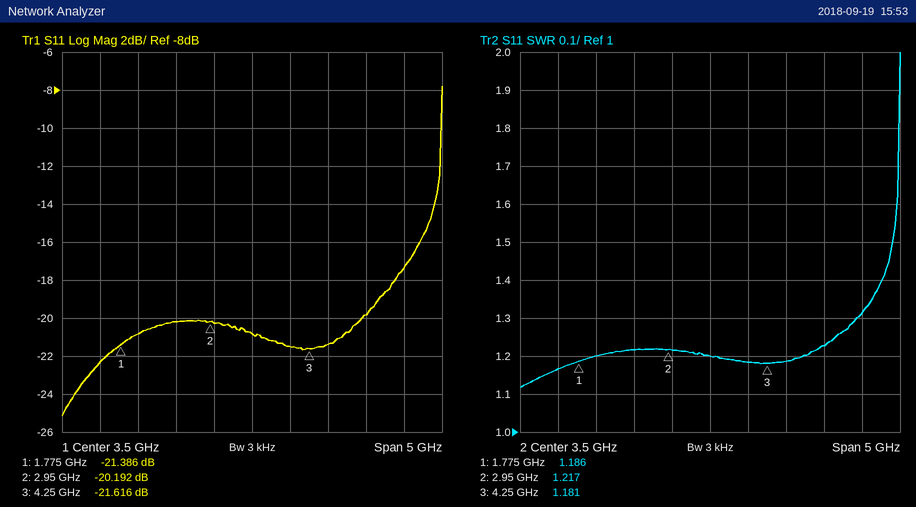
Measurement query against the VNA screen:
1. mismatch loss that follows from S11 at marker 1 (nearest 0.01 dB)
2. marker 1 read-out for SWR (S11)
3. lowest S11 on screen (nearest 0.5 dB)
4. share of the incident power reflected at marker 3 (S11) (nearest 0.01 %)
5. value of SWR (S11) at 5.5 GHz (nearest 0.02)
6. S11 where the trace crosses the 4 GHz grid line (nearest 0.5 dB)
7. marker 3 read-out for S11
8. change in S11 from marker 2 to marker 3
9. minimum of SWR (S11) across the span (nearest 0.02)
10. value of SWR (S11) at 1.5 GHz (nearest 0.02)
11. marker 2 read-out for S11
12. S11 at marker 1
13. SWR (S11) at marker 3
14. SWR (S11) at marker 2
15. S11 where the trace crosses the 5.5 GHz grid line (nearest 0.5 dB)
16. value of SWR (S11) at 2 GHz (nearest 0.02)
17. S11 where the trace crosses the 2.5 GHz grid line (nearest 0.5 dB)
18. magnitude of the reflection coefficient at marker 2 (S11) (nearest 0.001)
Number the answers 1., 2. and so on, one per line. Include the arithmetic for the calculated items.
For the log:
1. −10 log10(1 − 10^(-21.386/10)) ≈ 0.03 dB
2. 1.186
3. -25.0 dB
4. 10^(-21.616/10) ≈ 0.69 %
5. 1.32
6. -21.5 dB
7. -21.616 dB
8. -21.616 − (-20.192) = -1.424 dB
9. 1.12
10. 1.16
11. -20.192 dB
12. -21.386 dB
13. 1.181
14. 1.217
15. -17.5 dB
16. 1.20
17. -20.0 dB
18. 10^(-20.192/20) ≈ 0.098
